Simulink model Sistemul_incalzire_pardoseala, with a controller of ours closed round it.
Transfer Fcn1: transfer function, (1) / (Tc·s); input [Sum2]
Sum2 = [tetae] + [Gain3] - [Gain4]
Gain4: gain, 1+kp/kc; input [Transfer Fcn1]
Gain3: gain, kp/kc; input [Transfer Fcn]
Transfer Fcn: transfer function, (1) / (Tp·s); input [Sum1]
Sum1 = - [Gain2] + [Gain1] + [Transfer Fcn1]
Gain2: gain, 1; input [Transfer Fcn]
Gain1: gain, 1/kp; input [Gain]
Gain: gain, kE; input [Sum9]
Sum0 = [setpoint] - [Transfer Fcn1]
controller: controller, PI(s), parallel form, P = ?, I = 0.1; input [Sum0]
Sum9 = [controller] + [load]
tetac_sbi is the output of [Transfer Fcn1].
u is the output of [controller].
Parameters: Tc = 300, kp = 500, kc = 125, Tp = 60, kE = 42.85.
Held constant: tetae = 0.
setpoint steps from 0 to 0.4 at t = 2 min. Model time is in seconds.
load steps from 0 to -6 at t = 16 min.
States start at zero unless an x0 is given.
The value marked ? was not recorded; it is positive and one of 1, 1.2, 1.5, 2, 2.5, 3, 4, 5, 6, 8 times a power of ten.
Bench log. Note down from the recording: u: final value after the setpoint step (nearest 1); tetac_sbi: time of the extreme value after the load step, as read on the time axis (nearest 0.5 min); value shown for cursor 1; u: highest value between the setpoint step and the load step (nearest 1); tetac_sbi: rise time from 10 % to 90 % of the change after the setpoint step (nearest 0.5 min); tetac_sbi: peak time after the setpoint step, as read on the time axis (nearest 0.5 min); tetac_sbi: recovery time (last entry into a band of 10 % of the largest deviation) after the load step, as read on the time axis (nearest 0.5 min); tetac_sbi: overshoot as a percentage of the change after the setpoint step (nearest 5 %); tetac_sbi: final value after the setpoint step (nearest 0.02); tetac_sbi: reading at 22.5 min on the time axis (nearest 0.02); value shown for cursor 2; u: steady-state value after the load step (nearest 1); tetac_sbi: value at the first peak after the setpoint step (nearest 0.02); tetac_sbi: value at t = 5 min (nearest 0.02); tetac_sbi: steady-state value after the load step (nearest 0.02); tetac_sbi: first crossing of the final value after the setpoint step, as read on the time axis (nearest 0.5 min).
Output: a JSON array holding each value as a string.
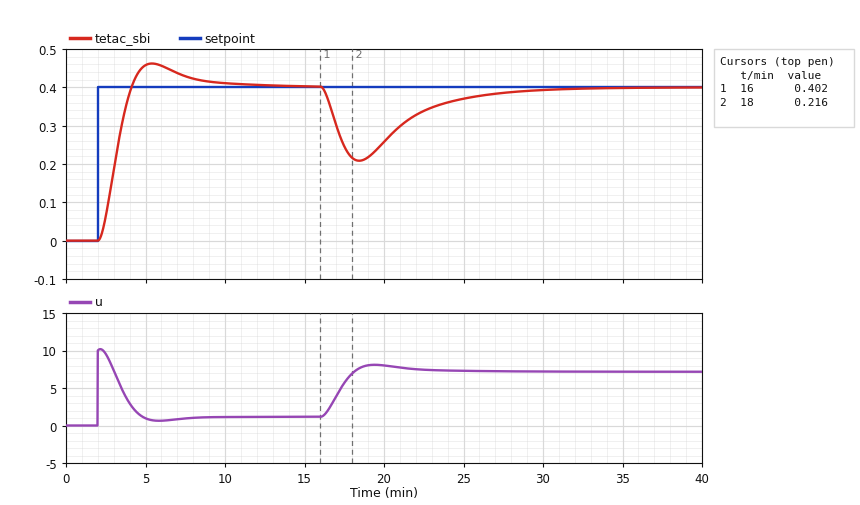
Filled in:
["1", "18.5 min", "0.402", "10", "1.5 min", "5.5 min", "26.5 min", "15 %", "0.40", "0.34", "0.216", "7", "0.46", "0.46", "0.40", "4.0 min"]
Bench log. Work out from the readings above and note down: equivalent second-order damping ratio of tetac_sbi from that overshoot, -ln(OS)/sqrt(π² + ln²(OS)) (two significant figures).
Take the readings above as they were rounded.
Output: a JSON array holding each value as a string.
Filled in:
["0.52"]
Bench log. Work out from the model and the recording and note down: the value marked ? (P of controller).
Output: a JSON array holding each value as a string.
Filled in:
["25"]
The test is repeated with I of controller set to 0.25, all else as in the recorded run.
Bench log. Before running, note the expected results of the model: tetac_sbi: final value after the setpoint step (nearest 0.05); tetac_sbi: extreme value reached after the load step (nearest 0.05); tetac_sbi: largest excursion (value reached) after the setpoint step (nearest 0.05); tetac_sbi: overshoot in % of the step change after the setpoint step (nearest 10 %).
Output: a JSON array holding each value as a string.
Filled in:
["0.40", "0.25", "0.55", "40 %"]
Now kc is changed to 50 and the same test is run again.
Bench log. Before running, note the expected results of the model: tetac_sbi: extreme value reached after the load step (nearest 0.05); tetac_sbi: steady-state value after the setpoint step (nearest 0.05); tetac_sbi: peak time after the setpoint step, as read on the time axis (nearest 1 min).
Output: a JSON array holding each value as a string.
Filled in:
["0.20", "0.40", "4 min"]
